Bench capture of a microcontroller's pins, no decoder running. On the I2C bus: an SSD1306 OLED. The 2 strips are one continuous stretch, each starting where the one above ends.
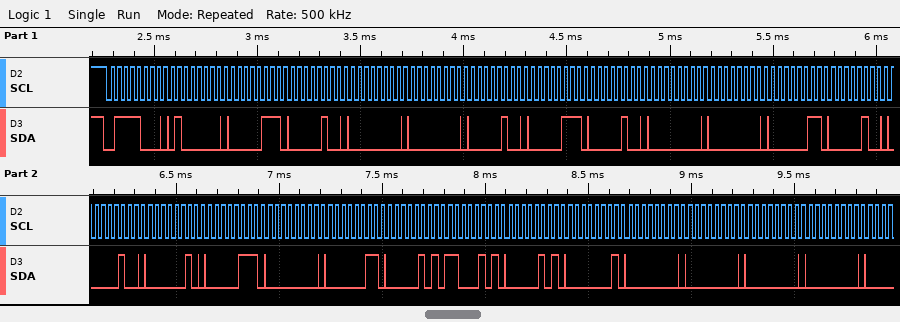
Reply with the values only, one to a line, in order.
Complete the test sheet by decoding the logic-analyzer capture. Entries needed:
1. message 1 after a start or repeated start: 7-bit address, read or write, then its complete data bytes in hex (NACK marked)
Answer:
0x3C write: 40 07 04 00 00 04 07 04 00 00 03 04 04 02 07 00 03 05 C5 05 01 00 00 00 00
